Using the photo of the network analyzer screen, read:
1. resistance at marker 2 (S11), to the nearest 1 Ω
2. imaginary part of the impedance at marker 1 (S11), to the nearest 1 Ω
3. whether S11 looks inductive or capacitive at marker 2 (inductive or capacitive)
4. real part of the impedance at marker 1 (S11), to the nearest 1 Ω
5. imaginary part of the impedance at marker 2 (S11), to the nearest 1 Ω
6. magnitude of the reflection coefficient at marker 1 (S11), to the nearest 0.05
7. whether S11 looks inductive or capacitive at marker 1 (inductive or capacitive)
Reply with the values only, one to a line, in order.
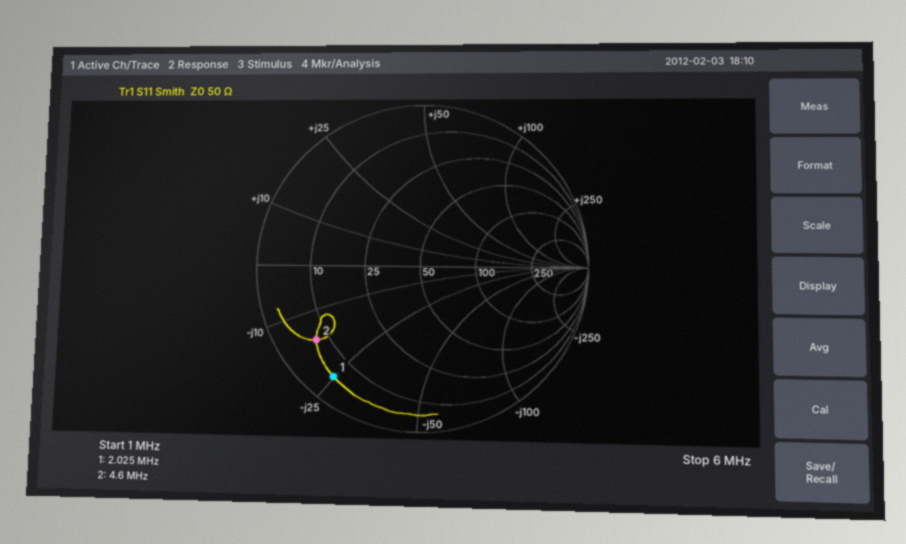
7 Ω
-25 Ω
capacitive
5 Ω
-16 Ω
0.85
capacitive
